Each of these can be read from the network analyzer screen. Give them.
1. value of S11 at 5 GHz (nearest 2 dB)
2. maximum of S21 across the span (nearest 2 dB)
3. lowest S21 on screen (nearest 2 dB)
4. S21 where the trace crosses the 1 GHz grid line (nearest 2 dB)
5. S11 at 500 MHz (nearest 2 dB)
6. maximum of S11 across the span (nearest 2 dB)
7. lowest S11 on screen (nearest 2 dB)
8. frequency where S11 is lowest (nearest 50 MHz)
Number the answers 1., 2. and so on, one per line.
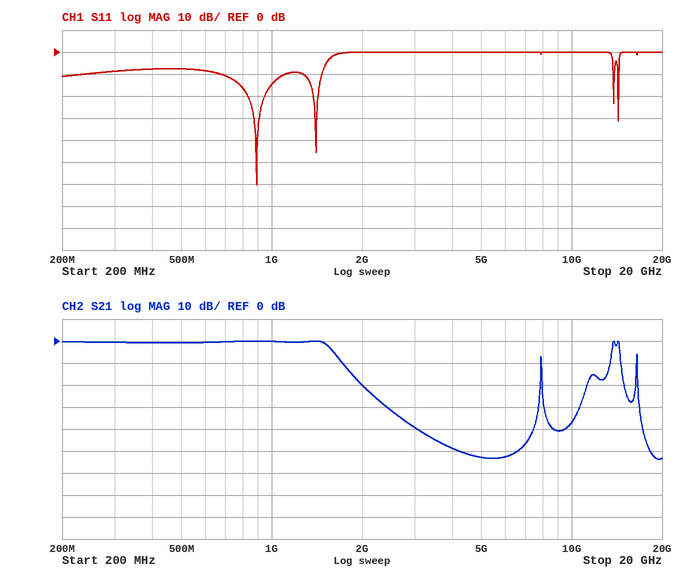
1. 0 dB
2. 0 dB
3. -54 dB
4. 0 dB
5. -8 dB
6. 0 dB
7. -60 dB
8. 900 MHz
